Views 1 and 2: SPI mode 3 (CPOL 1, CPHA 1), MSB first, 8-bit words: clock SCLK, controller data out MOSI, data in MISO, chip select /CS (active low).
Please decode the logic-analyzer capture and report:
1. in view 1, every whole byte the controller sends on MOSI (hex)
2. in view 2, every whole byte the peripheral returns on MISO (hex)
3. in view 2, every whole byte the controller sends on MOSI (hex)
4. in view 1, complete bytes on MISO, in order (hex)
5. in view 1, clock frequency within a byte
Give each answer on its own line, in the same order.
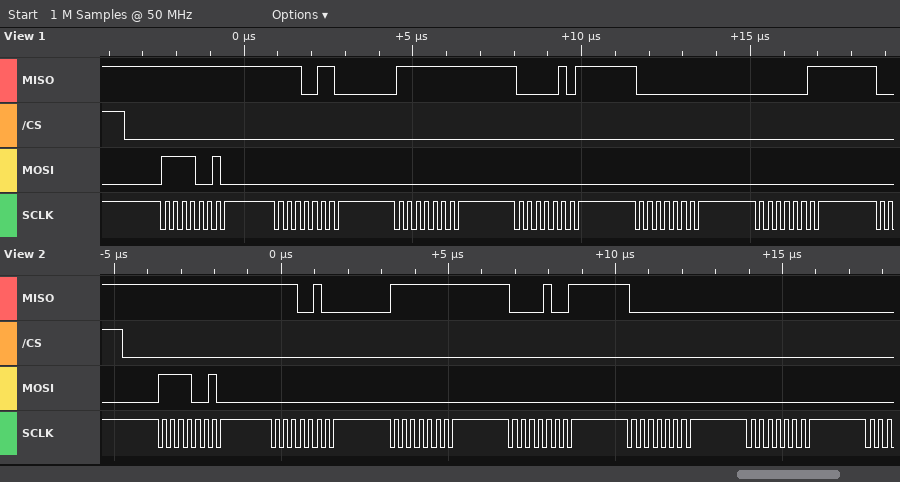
F2 00 00 00 00 00
FF E4 FF 09 00 00
F2 00 00 00 00 00
FF E6 FF 05 00 03
4 MHz
